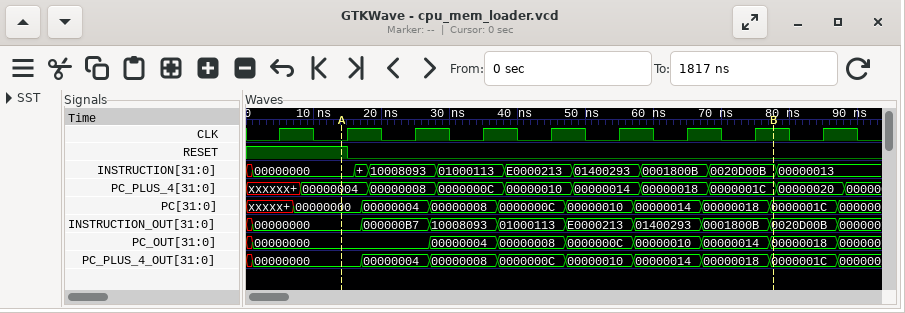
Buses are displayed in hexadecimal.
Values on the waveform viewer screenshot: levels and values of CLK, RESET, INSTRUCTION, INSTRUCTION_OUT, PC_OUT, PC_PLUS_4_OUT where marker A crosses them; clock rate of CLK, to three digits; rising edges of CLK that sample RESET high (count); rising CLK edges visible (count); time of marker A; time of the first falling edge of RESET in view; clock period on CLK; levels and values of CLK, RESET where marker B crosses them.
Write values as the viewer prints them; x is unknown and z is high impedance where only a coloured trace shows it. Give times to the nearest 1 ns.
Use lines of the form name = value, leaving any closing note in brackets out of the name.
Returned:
levels and values of CLK, RESET, INSTRUCTION, INSTRUCTION_OUT, PC_OUT, PC_PLUS_4_OUT where marker A crosses them = CLK=0, RESET=1, INSTRUCTION=00000000, INSTRUCTION_OUT=00000000, PC_OUT=00000000, PC_PLUS_4_OUT=00000000
clock rate of CLK, to three digits = 100 MHz
rising edges of CLK that sample RESET high = 2
rising CLK edges visible = 9
time of marker A = 14 ns
time of the first falling edge of RESET in view = 15 ns
clock period on CLK = 10 ns
levels and values of CLK, RESET where marker B crosses them = CLK=1, RESET=0
